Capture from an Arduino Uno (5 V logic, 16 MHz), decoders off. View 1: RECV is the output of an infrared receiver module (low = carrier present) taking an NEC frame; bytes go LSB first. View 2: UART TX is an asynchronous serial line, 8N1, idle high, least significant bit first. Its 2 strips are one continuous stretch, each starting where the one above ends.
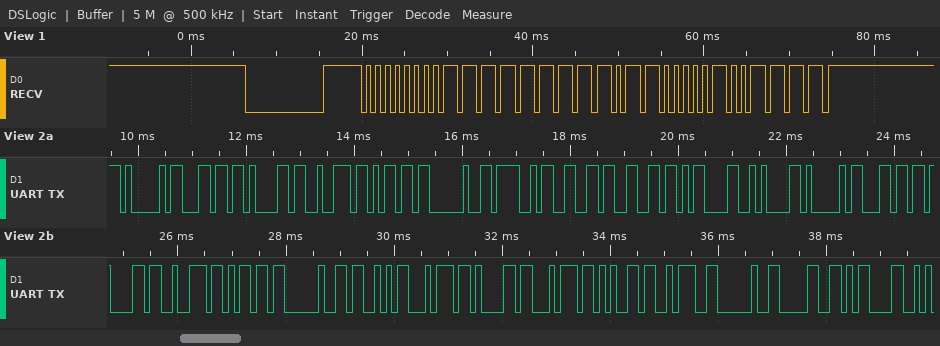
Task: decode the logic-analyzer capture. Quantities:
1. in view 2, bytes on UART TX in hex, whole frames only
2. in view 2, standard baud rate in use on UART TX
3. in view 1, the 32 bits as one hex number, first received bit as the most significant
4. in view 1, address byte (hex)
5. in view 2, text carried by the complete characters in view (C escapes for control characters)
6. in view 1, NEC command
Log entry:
41 6C 61 72 6D 20 4F 66 66 0D 0A 41 6C 61 72 6D 20 53 74 61 74 65 3A 20 30 0D
9600 baud
0x00FFB04F
0x00
"Alarm Off\r\nAlarm State: 0\r"
0x0D
